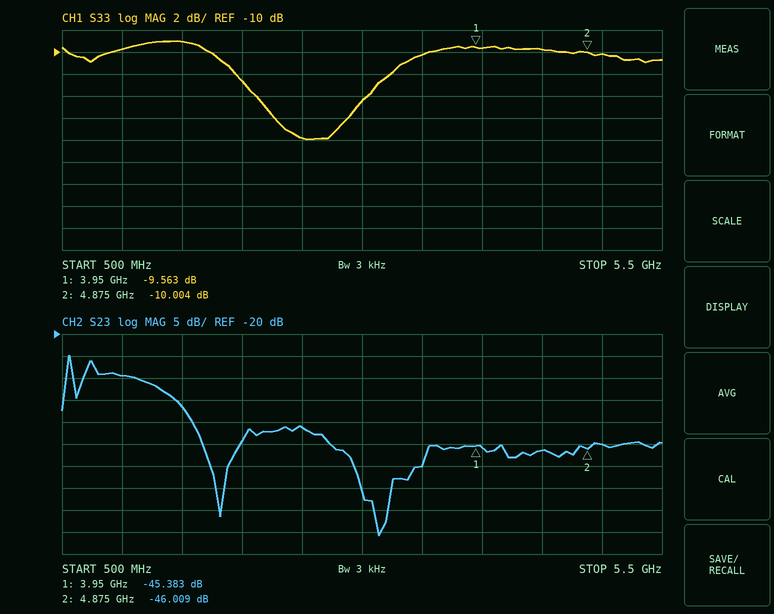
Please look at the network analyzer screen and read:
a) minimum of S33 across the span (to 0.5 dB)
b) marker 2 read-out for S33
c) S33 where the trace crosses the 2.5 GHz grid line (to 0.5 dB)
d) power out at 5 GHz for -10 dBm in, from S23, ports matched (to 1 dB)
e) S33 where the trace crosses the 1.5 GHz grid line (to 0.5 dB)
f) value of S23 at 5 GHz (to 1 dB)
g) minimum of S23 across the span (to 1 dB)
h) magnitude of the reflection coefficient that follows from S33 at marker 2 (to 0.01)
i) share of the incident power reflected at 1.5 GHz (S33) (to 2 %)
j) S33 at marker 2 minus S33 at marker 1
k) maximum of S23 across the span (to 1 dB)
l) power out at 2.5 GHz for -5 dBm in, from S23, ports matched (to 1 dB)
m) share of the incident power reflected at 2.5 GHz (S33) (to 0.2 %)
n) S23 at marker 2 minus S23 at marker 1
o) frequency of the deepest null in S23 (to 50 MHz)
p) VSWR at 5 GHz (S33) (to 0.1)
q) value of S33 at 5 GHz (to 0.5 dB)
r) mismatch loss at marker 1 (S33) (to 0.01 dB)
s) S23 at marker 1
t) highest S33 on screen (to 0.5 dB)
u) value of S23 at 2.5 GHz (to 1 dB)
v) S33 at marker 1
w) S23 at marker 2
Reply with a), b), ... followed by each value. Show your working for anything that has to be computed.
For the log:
a) -18.0 dB
b) -10.004 dB
c) -18.0 dB
d) -10 dBm + (-45 dB) = -55 dBm
e) -9.0 dB
f) -45 dB
g) -66 dB
h) 10^(-10.004/20) ≈ 0.32
i) 10^(-9/10) ≈ 12.6 %, so 12 % to the nearest 2 %
j) -10.004 − (-9.563) = -0.441 dB
k) -25 dB
l) -5 dBm + (-41 dB) = -46 dBm
m) 10^(-18/10) ≈ 1.6 %
n) -46.009 − (-45.383) = -0.626 dB
o) 3.15 GHz
p) |Γ| = 10^(-10/20) = 0.3162; VSWR = (1 + 0.3162)/(1 − 0.3162) ≈ 1.9
q) -10.0 dB
r) −10 log10(1 − 10^(-9.563/10)) ≈ 0.51 dB
s) -45.383 dB
t) -9.0 dB
u) -41 dB
v) -9.563 dB
w) -46.009 dB
